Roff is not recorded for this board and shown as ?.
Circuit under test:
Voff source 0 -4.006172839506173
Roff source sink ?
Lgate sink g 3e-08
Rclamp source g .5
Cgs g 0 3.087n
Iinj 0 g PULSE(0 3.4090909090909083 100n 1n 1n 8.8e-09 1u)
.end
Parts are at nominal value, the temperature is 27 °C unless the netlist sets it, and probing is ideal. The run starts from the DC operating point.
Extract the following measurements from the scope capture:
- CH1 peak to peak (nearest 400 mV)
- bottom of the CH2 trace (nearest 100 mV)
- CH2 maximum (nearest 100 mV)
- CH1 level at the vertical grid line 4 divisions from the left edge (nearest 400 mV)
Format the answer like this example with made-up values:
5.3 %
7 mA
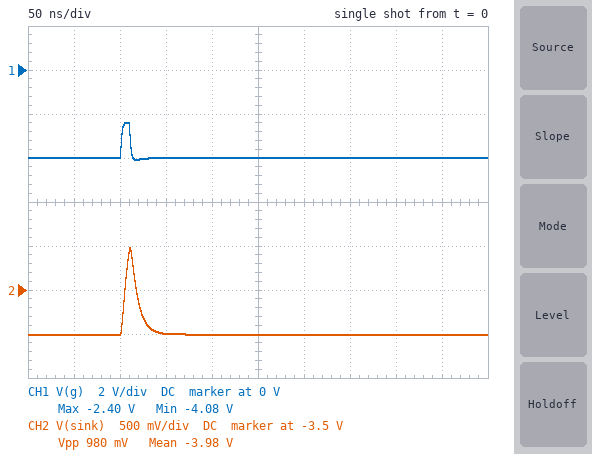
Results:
1.6 V
-4.0 V
-3.0 V
-4.0 V
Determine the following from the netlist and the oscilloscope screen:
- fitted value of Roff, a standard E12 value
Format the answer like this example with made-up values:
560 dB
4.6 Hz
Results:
3.3 Ω
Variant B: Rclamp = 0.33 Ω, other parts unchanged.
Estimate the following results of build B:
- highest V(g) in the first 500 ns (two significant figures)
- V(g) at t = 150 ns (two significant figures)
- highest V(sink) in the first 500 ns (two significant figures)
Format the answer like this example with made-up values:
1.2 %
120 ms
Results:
-2.9 V
-4.0 V
-3.3 V
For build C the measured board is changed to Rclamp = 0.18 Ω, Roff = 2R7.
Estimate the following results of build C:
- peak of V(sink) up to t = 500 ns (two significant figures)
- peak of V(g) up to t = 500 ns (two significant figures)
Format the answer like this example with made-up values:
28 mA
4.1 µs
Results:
-3.7 V
-3.4 V
